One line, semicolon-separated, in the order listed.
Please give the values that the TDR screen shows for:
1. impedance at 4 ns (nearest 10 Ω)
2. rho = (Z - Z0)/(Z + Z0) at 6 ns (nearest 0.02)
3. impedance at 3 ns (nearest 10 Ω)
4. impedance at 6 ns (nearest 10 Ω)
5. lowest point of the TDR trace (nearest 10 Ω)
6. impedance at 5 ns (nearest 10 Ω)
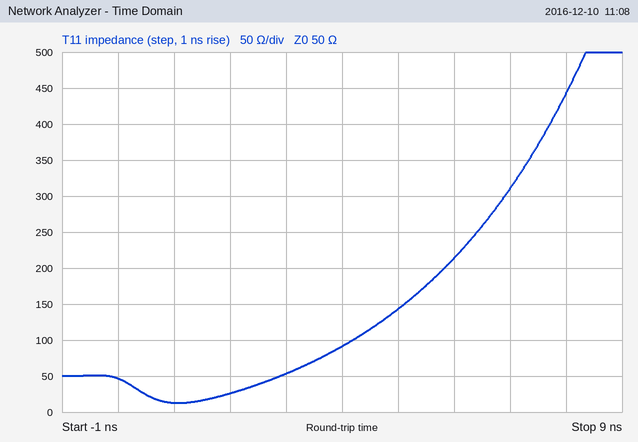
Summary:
90 Ω; +0.62; 50 Ω; 210 Ω; 10 Ω; 140 Ω
